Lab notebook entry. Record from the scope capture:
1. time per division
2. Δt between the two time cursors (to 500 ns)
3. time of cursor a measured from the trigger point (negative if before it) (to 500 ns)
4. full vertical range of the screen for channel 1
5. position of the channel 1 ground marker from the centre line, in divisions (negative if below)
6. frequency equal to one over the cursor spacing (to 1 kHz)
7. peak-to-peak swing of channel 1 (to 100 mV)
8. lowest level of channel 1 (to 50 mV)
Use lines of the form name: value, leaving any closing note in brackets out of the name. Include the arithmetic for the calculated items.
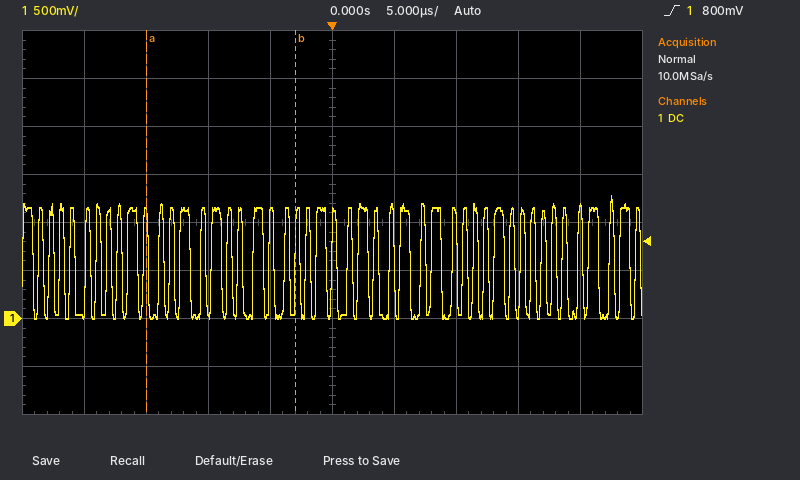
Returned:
time per division: 5 µs
Δt between the two time cursors: 12.0 µs
time of cursor a measured from the trigger point (negative if before it): -15.0 µs
full vertical range of the screen for channel 1: 4 V
position of the channel 1 ground marker from the centre line, in divisions: -2.0 div
frequency equal to one over the cursor spacing: 1 / 12.0 µs ≈ 83 kHz
peak-to-peak swing of channel 1: 1.30 V
lowest level of channel 1: 0 mV
